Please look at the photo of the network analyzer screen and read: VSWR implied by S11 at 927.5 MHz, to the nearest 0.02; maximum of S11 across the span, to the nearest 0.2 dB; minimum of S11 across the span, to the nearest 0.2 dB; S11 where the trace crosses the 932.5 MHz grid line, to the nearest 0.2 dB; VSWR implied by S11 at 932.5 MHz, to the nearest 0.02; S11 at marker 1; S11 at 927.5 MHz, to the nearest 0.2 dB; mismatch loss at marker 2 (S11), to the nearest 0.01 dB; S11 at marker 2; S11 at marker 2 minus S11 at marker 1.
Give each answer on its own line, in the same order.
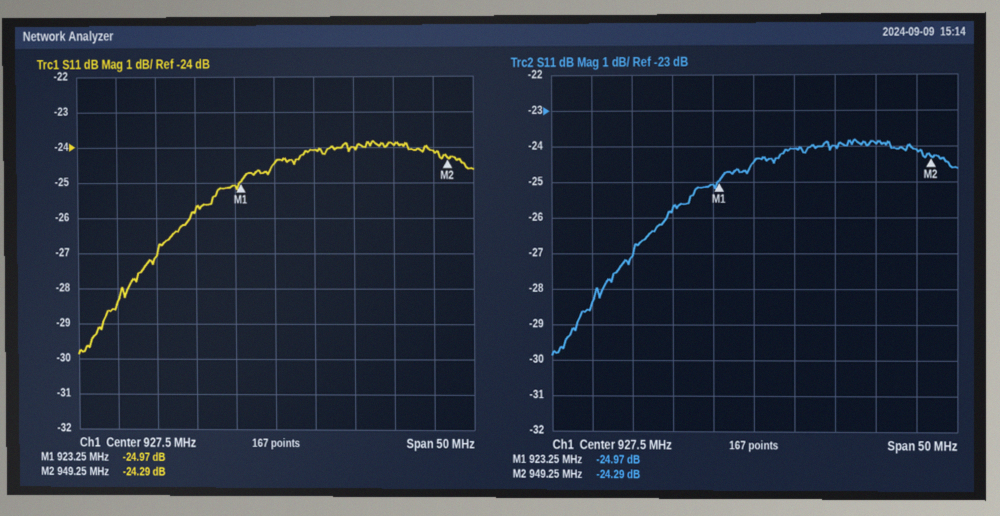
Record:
1.12
-23.8 dB
-29.8 dB
-24.0 dB
1.14
-24.97 dB
-24.4 dB
0.02 dB
-24.29 dB
0.68 dB
